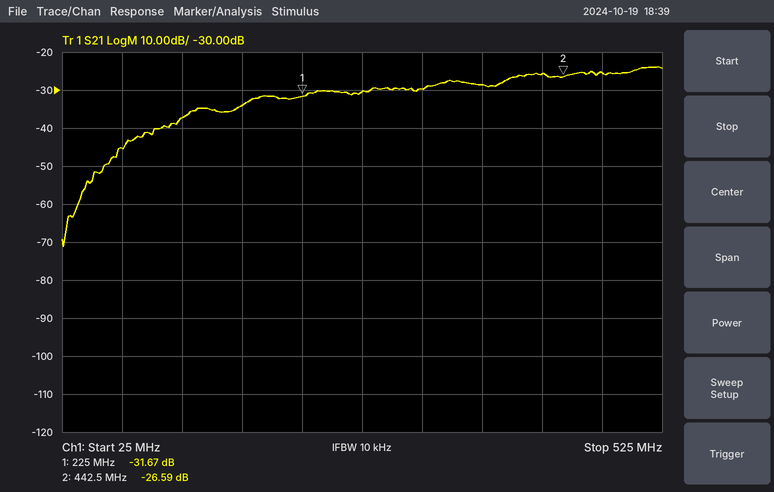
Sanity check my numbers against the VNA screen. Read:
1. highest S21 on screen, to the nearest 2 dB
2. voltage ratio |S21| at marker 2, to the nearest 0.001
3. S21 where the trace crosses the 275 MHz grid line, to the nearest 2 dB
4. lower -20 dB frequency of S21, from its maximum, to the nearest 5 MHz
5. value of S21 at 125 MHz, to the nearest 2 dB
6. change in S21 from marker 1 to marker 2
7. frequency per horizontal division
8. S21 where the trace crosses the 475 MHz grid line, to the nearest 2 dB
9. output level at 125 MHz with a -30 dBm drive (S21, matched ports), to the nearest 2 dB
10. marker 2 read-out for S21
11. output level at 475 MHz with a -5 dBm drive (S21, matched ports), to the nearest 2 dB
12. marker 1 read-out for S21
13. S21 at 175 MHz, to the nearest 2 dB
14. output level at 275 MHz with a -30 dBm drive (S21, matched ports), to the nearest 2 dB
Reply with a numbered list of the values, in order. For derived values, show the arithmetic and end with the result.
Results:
1. -24 dB
2. 10^(-26.59/20) ≈ 0.047
3. -30 dB
4. 80 MHz
5. -38 dB
6. -26.59 − (-31.67) = 5.08 dB
7. 50 MHz
8. -26 dB
9. -30 dBm + (-38 dB) = -68 dBm
10. -26.59 dB
11. -5 dBm + (-26 dB) = -30 dBm
12. -31.67 dB
13. -34 dB
14. -30 dBm + (-30 dB) = -60 dBm
